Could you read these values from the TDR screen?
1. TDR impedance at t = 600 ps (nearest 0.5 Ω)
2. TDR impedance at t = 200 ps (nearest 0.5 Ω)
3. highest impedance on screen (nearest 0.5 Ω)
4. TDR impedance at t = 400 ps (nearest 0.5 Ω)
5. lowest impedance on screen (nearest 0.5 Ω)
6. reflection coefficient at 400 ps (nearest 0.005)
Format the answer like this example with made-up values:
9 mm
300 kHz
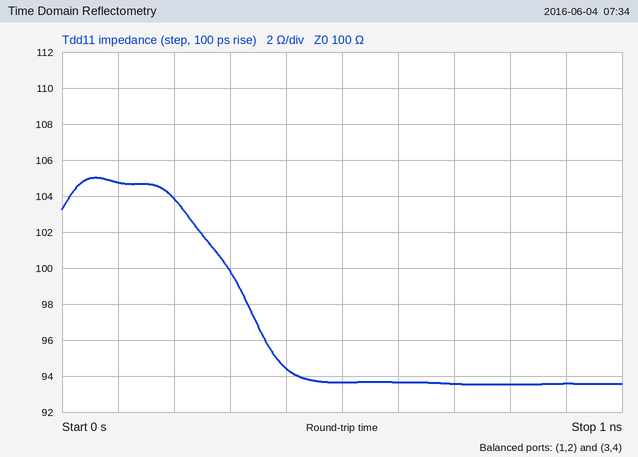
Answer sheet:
93.5 Ω
104.0 Ω
105.0 Ω
94.5 Ω
93.5 Ω
-0.030
